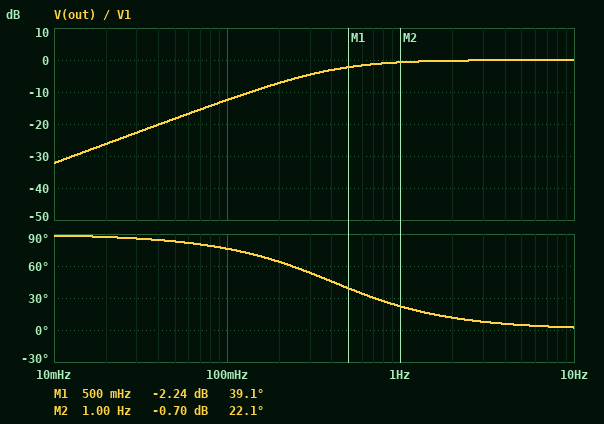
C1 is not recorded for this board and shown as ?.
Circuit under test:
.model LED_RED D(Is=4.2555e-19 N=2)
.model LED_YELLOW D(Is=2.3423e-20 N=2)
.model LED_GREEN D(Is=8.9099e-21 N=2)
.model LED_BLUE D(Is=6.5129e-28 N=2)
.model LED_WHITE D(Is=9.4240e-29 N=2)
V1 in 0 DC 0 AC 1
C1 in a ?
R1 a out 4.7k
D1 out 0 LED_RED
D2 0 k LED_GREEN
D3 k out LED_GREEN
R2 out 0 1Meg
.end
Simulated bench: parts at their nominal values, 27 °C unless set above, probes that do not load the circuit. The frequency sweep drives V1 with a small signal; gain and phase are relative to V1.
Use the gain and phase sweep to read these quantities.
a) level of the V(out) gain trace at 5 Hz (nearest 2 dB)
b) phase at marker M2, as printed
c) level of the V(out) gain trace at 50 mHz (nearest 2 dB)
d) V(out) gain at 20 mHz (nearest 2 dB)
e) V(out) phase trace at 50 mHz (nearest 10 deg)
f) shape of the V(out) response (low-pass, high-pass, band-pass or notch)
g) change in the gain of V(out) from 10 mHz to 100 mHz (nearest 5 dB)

0 dB
22.1 deg
-18 dB
-26 dB
80 deg
high-pass
20 dB
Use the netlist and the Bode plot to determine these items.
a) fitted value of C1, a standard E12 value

390 nF
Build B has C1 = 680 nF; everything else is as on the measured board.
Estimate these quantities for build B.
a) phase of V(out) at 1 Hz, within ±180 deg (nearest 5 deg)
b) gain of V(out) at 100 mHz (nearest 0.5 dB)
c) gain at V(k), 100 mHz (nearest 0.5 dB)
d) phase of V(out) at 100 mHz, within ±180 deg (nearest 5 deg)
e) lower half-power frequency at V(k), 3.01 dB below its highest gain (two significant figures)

15 deg
-8.0 dB
-14.0 dB
65 deg
230 mHz
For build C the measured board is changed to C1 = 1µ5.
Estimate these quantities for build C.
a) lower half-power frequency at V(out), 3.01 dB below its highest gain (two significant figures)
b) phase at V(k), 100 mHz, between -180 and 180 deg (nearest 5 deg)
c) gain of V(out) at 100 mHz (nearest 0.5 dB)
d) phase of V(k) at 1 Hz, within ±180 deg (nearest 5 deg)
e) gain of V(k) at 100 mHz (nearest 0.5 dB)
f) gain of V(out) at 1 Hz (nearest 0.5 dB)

110 mHz
45 deg
-3.5 dB
5 deg
-9.5 dB
0 dB
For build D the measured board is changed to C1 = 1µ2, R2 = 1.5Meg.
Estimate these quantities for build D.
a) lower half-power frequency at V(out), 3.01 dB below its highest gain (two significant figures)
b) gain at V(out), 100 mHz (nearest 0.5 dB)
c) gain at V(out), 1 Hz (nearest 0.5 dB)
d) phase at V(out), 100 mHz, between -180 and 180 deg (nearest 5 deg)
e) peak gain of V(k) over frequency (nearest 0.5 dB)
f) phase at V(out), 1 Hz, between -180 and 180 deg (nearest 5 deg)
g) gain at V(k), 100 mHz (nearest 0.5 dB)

88 mHz
-2.5 dB
0 dB
40 deg
-6.0 dB
5 deg
-8.5 dB
